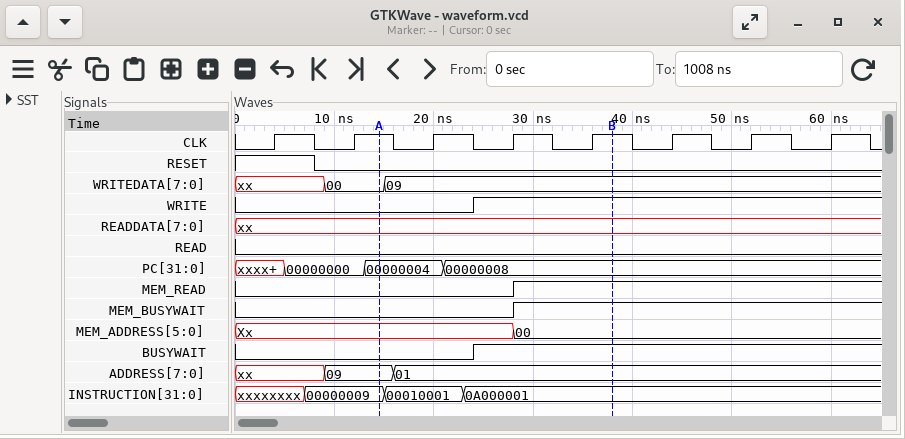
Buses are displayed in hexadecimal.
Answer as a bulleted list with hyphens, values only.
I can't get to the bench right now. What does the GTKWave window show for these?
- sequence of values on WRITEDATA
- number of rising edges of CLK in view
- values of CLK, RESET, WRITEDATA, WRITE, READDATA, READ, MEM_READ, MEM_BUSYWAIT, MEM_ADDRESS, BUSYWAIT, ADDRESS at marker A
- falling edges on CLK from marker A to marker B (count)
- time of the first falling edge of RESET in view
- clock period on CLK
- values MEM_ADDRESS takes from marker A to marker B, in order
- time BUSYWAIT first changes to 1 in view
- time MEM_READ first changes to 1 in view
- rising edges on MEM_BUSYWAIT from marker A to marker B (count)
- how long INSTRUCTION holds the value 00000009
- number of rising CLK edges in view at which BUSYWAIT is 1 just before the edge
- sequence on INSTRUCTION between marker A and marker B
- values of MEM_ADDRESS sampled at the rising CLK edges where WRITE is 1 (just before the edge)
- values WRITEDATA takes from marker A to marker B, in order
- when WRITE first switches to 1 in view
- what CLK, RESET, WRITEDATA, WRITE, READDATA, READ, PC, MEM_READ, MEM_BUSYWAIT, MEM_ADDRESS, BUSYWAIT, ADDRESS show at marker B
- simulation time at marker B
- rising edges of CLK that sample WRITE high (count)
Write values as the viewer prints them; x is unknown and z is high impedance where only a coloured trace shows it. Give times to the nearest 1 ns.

- xx, 00, 09
- 8
- CLK=1, RESET=0, WRITEDATA=00, WRITE=0, READDATA=xx, READ=0, MEM_READ=0, MEM_BUSYWAIT=0, MEM_ADDRESS=Xx, BUSYWAIT=0, ADDRESS=09
- 3
- 8 ns
- 8 ns
- Xx, 00
- 24 ns
- 28 ns
- 1
- 8 ns
- 5
- 00000009, 00010001, 0A000001
- Xx, 00, 00, 00, 00
- 00, 09
- 24 ns
- CLK=1, RESET=0, WRITEDATA=09, WRITE=1, READDATA=xx, READ=0, PC=00000008, MEM_READ=1, MEM_BUSYWAIT=1, MEM_ADDRESS=00, BUSYWAIT=1, ADDRESS=01
- 38 ns
- 5
